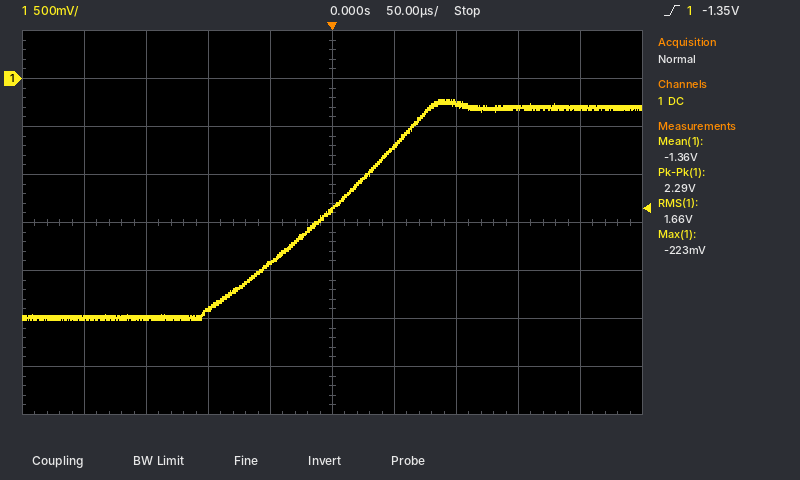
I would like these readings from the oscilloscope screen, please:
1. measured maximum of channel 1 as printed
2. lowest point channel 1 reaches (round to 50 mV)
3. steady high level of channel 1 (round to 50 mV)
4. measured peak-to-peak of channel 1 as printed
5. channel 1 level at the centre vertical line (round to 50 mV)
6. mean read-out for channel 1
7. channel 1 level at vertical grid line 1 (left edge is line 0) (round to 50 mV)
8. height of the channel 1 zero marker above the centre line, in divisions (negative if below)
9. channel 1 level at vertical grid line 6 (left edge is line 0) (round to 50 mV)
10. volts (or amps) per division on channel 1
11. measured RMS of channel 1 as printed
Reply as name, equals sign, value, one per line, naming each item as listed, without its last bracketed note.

measured maximum of channel 1 as printed = -223 mV
lowest point channel 1 reaches = -2.50 V
steady high level of channel 1 = -300 mV
measured peak-to-peak of channel 1 as printed = 2.29 V
channel 1 level at the centre vertical line = -1.35 V
mean read-out for channel 1 = -1.36 V
channel 1 level at vertical grid line 1 (left edge is line 0) = -2.50 V
height of the channel 1 zero marker above the centre line, in divisions = +3.0 div
channel 1 level at vertical grid line 6 (left edge is line 0) = -700 mV
volts (or amps) per division on channel 1 = 500 mV
measured RMS of channel 1 as printed = 1.66 V
